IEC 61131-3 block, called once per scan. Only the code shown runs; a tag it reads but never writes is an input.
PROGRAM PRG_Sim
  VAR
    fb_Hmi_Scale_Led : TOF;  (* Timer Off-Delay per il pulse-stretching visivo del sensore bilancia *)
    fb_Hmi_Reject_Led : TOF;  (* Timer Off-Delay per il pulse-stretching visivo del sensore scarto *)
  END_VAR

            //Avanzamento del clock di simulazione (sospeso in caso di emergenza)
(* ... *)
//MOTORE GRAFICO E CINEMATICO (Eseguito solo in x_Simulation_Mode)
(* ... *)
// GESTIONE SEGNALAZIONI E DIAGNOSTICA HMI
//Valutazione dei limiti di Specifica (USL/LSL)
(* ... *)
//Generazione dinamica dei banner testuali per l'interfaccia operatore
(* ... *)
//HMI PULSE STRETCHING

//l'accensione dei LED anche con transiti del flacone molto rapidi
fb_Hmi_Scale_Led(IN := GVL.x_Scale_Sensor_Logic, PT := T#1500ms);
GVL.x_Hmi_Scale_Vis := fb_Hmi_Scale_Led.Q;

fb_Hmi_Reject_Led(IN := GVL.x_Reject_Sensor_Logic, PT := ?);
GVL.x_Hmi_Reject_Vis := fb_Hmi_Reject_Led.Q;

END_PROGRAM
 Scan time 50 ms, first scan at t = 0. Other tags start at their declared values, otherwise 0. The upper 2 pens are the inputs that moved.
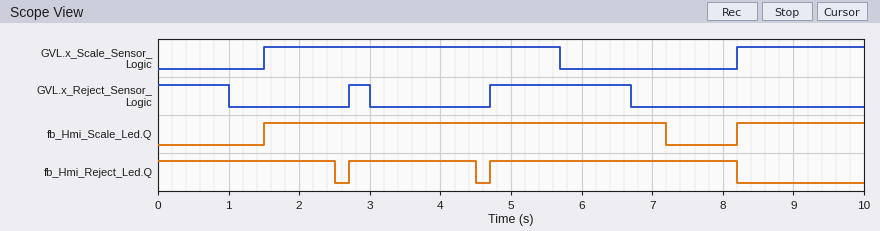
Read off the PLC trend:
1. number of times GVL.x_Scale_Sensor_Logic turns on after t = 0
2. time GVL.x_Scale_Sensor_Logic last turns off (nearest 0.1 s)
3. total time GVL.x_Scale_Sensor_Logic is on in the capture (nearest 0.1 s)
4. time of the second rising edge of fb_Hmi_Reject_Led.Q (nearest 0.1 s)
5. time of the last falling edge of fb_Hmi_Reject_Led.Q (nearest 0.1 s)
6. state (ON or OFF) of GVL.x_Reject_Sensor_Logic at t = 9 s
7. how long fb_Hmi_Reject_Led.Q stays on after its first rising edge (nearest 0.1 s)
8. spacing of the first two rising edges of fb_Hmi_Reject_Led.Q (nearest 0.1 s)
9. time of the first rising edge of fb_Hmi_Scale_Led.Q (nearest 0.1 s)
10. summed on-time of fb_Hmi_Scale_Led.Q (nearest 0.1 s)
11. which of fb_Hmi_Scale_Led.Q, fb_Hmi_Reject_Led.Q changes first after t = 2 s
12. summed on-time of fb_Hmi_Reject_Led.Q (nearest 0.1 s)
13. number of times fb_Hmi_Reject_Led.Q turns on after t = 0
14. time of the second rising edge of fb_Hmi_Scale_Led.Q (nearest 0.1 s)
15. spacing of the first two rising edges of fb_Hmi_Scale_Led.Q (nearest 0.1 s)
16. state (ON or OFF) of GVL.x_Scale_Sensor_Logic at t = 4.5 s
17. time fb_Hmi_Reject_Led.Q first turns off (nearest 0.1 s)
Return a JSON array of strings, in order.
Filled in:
["2", "5.7 s", "6.0 s", "4.7 s", "8.2 s", "OFF", "1.8 s", "2.0 s", "1.5 s", "7.5 s", "fb_Hmi_Reject_Led.Q", "7.8 s", "2", "8.2 s", "6.7 s", "ON", "2.5 s"]
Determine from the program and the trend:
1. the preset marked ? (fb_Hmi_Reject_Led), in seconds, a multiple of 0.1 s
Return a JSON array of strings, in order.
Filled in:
["1.5 s"]
